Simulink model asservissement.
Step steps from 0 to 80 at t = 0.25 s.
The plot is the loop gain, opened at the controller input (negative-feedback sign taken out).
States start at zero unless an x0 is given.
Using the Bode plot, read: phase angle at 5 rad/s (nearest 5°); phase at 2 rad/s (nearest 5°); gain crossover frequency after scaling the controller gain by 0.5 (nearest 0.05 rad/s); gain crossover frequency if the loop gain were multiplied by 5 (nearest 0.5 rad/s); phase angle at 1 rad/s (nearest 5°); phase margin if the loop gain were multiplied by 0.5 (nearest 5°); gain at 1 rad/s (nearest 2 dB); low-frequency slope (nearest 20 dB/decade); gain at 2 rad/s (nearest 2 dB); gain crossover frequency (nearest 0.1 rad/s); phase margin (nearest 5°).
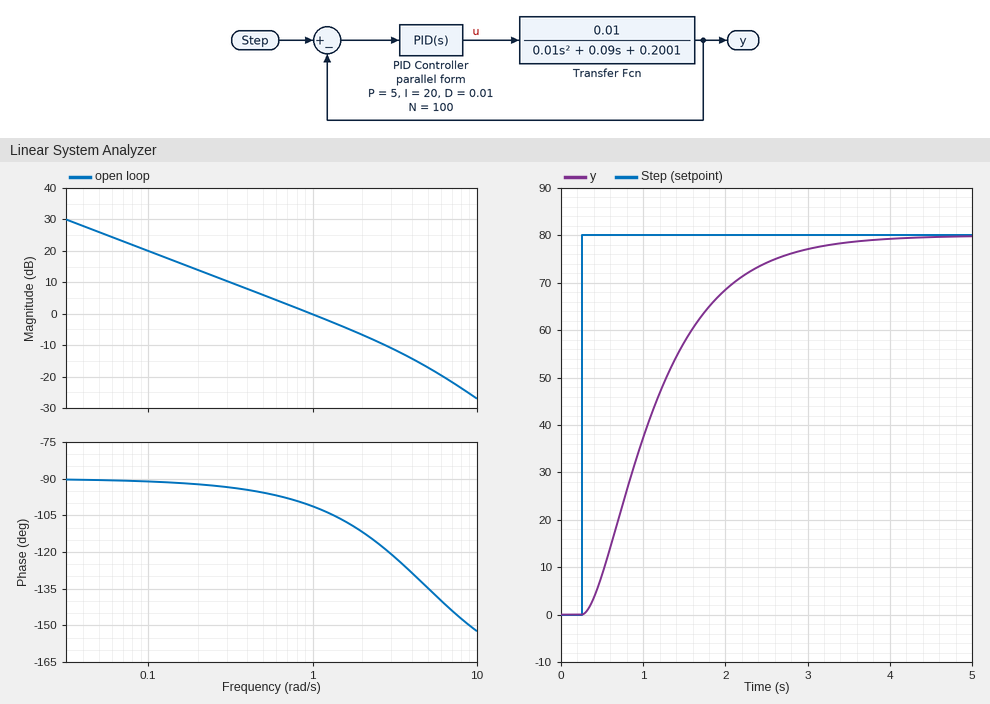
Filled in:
-135°
-110°
0.50 rad/s
4.0 rad/s
-100°
85°
0 dB
-20 dB/decade
-6 dB
1.0 rad/s
80°
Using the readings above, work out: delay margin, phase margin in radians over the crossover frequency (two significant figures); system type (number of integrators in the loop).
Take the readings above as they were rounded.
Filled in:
1.4 s
1
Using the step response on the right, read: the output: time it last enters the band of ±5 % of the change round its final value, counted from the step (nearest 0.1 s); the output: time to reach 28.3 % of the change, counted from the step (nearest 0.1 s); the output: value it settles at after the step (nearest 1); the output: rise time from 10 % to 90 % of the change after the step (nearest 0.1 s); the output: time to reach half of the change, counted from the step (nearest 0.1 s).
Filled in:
2.5 s
0.5 s
80
1.8 s
0.8 s
